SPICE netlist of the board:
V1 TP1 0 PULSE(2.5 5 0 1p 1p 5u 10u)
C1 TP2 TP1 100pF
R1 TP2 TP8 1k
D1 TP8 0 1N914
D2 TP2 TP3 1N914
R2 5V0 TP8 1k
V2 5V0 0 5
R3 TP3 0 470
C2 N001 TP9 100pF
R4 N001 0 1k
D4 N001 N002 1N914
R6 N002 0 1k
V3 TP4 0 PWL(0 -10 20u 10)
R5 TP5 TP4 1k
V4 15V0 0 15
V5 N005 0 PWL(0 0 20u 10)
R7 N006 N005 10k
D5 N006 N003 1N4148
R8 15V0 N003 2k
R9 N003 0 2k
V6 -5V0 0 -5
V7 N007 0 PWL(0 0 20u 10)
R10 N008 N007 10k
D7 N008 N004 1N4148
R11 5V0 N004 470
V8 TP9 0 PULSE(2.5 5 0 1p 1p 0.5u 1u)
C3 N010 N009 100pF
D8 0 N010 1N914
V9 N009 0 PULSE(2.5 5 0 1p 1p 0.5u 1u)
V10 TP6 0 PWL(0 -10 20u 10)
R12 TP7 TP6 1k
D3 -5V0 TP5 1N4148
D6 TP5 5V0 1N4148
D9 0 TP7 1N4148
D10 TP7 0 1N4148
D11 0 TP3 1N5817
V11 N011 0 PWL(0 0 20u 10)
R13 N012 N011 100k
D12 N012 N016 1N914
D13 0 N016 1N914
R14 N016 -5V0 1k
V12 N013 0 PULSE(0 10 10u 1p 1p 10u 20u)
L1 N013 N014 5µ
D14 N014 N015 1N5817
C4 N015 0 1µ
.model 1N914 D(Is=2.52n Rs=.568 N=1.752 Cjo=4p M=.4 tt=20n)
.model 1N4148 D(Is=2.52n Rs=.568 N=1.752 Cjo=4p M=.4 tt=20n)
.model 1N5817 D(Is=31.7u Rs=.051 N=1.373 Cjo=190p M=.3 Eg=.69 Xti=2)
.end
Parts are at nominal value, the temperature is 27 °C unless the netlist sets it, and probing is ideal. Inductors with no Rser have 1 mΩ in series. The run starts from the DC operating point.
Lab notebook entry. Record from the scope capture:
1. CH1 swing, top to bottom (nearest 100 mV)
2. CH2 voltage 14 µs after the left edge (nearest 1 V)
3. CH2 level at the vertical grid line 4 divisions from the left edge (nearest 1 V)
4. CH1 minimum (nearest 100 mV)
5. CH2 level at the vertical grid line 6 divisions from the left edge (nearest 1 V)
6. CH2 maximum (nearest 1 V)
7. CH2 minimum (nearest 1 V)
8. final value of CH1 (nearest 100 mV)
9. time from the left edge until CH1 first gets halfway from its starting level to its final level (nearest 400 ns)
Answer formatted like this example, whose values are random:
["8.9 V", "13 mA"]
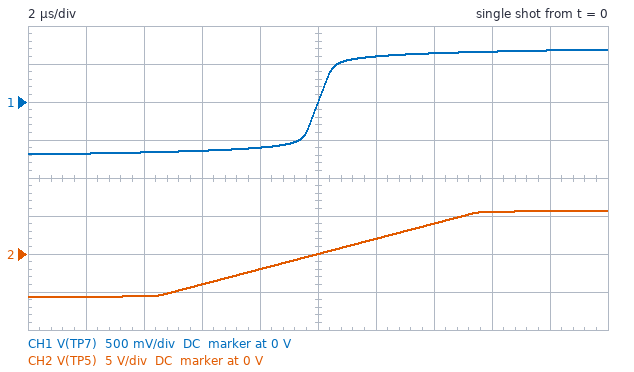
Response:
["1.4 V", "4 V", "-2 V", "-700 mV", "2 V", "6 V", "-6 V", "700 mV", "10.0 µs"]
